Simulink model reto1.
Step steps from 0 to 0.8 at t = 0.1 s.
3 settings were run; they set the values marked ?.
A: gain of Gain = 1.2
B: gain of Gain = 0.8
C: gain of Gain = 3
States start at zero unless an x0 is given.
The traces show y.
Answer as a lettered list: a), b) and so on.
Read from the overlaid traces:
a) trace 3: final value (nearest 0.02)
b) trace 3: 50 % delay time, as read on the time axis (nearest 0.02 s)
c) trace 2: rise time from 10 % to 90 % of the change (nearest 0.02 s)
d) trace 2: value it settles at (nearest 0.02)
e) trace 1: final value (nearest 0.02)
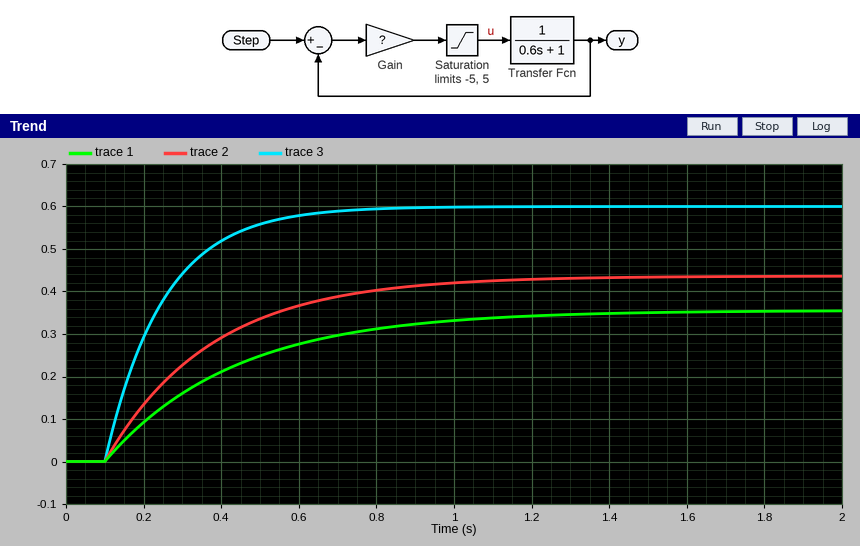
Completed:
a) 0.60
b) 0.20 s
c) 0.60 s
d) 0.44
e) 0.36
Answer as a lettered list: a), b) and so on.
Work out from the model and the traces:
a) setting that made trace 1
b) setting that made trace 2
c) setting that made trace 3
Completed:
a) B
b) A
c) C
